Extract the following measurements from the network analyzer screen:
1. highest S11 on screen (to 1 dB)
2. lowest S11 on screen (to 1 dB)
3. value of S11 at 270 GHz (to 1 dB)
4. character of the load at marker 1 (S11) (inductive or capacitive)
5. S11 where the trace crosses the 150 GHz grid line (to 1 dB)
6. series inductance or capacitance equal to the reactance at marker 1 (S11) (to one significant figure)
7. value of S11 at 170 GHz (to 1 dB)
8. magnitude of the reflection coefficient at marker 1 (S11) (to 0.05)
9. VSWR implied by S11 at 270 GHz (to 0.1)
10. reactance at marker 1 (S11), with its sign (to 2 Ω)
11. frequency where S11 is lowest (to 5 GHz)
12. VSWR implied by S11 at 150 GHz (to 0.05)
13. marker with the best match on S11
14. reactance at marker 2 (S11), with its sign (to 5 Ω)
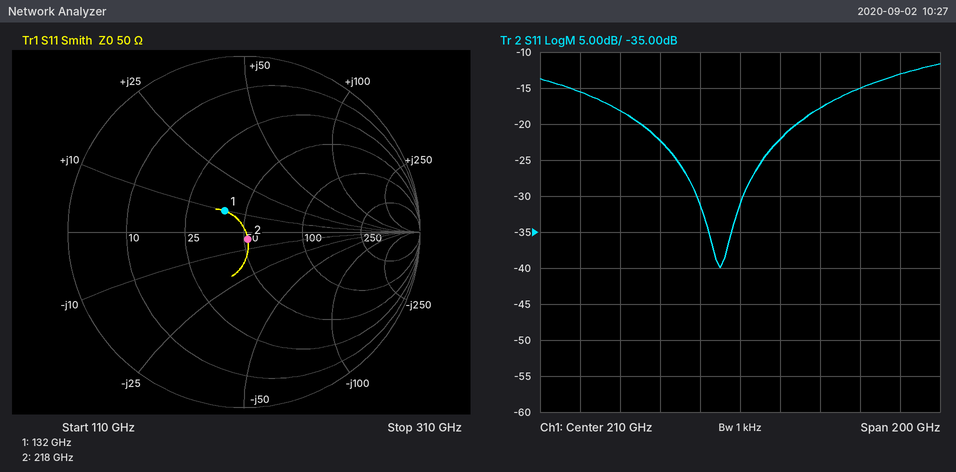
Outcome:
-12 dB
-40 dB
-15 dB
inductive
-18 dB
10 pH
-22 dB
0.15
1.4
+10 Ω
200 GHz
1.30
marker 2
-5 Ω
